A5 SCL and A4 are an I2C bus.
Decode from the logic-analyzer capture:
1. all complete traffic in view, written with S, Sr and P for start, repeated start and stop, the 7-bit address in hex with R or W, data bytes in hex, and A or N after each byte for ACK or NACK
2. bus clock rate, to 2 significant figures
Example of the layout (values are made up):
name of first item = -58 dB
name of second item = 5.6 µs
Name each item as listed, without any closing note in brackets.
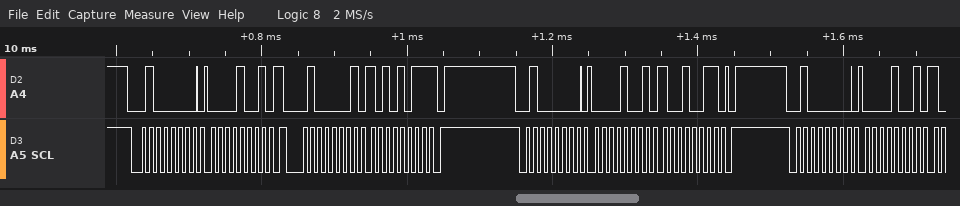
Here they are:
all complete traffic in view, written with S, Sr and P for start, repeated start and stop, the 7-bit address in hex with R or W, data bytes in hex, and A or N after each byte for ACK or NACK = S 20W A 09 A Sr 20R A AB N P S 20W A 09 A 93 A P S 20W A 09 A
bus clock rate, to 2 significant figures = 100 kHz
